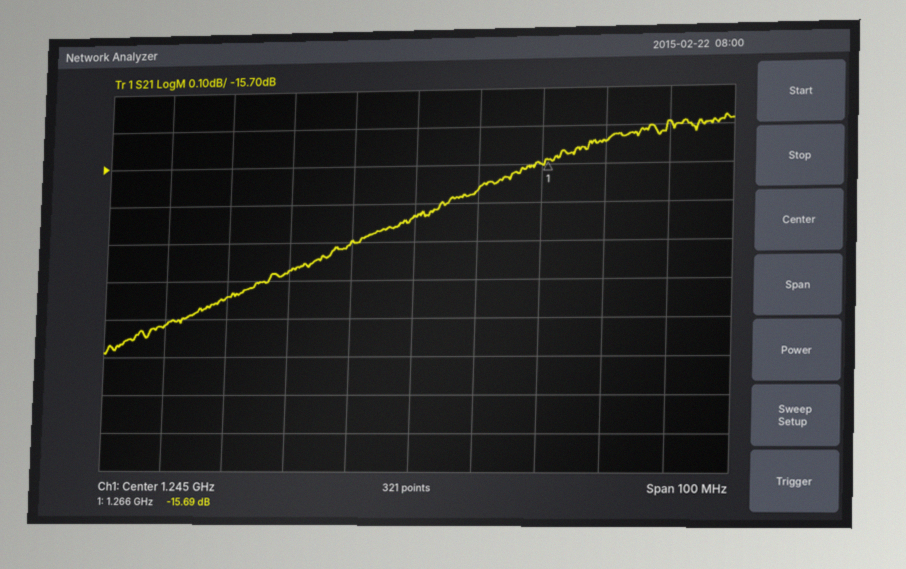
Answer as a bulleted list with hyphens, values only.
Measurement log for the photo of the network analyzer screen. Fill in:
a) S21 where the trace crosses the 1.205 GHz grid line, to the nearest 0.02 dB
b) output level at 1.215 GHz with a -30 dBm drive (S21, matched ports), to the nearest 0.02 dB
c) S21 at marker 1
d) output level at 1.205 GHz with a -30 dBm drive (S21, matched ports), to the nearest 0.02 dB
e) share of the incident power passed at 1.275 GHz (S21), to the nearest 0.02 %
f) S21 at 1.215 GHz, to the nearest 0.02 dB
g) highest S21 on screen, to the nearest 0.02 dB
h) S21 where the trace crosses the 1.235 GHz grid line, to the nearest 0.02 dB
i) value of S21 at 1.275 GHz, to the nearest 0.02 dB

- -16.12 dB
- -46.04 dBm
- -15.69 dB
- -46.12 dBm
- 2.72 %
- -16.04 dB
- -15.58 dB
- -15.90 dB
- -15.64 dB
